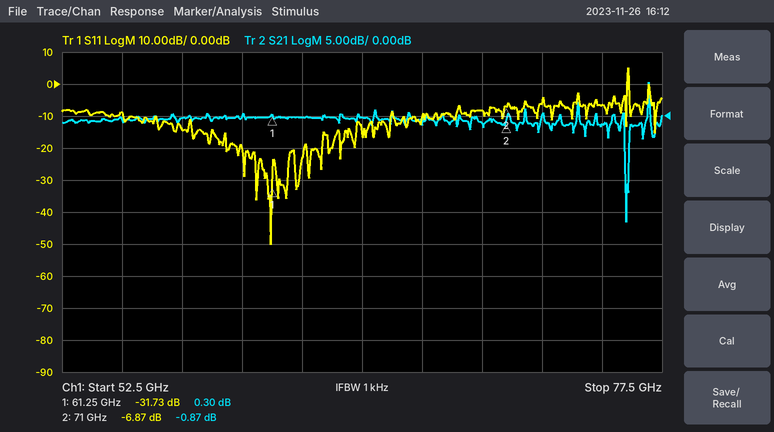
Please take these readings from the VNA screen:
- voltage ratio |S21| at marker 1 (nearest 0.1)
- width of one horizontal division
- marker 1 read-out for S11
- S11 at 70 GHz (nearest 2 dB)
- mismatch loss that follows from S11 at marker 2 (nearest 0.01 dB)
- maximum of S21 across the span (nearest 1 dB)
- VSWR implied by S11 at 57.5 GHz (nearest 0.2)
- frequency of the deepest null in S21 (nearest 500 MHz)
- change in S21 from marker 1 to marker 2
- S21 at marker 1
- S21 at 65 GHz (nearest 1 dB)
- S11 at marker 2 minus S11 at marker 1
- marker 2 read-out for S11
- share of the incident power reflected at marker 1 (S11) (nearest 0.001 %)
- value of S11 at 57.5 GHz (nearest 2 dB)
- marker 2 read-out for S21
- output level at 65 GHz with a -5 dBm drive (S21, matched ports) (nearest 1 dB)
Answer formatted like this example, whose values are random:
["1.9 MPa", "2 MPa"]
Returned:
["1.0", "2.5 GHz", "-31.73 dB", "-8 dB", "1.00 dB", "5 dB", "1.4", "76.0 GHz", "-1.17 dB", "0.30 dB", "0 dB", "24.86 dB", "-6.87 dB", "0.067 %", "-14 dB", "-0.87 dB", "-5 dBm"]
